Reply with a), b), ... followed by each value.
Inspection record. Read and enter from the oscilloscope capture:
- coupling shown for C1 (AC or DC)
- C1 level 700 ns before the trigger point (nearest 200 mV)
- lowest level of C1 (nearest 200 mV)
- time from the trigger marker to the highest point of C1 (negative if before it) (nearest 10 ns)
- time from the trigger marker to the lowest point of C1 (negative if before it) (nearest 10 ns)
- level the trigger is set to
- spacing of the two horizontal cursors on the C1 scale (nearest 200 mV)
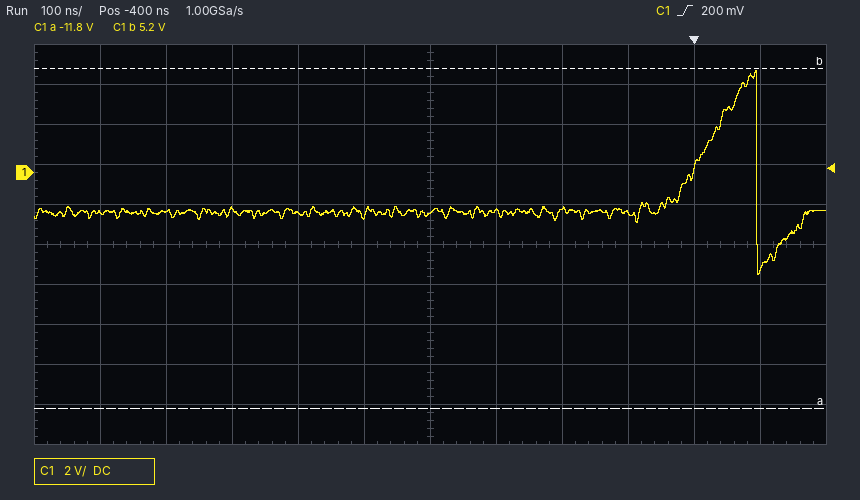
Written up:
a) DC
b) -1.8 V
c) -5.0 V
d) +90 ns
e) +100 ns
f) 200 mV
g) 17.0 V
